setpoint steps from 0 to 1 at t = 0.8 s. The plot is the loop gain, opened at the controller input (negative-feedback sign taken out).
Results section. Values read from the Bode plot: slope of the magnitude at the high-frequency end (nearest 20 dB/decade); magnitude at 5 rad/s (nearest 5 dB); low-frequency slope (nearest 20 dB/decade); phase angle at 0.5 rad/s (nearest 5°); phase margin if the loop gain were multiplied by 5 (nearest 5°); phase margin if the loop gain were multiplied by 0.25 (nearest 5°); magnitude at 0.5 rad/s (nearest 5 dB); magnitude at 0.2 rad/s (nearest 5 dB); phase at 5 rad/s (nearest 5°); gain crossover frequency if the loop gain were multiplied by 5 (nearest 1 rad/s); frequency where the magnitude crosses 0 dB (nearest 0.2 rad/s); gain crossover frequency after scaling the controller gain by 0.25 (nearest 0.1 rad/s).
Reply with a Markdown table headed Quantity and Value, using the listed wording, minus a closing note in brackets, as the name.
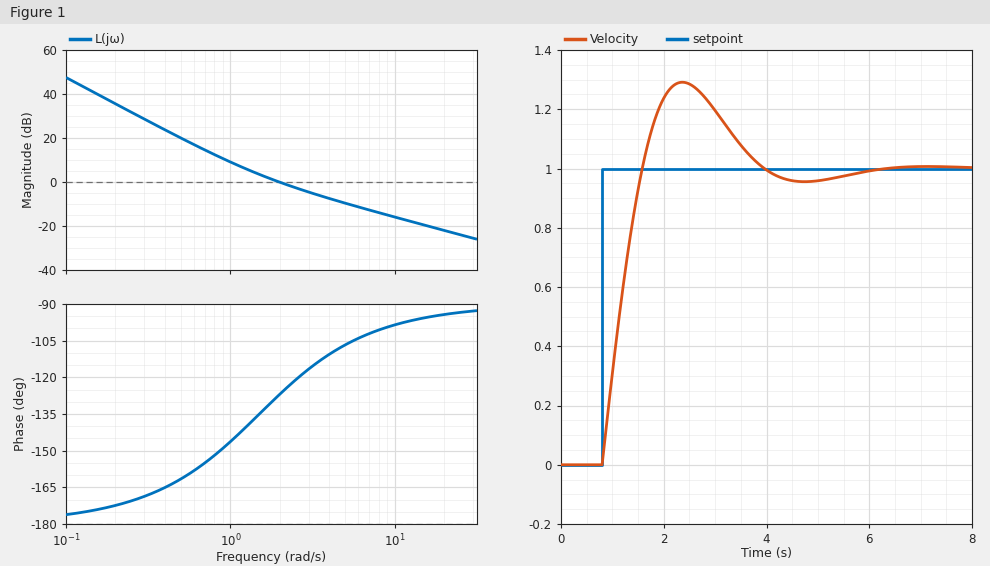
| Quantity | Value |
|---|---|
| slope of the magnitude at the high-frequency end | -20 dB/decade |
| magnitude at 5 rad/s | -10 dB |
| low-frequency slope | -40 dB/decade |
| phase angle at 0.5 rad/s | -160° |
| phase margin if the loop gain were multiplied by 5 | 80° |
| phase margin if the loop gain were multiplied by 0.25 | 30° |
| magnitude at 0.5 rad/s | 20 dB |
| magnitude at 0.2 rad/s | 35 dB |
| phase at 5 rad/s | -105° |
| gain crossover frequency if the loop gain were multiplied by 5 | 8 rad/s |
| frequency where the magnitude crosses 0 dB | 2.0 rad/s |
| gain crossover frequency after scaling the controller gain by 0.25 | 0.8 rad/s |
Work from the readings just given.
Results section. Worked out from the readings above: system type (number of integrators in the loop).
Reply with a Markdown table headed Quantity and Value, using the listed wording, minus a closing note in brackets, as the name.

| Quantity | Value |
|---|---|
| system type | 2 |
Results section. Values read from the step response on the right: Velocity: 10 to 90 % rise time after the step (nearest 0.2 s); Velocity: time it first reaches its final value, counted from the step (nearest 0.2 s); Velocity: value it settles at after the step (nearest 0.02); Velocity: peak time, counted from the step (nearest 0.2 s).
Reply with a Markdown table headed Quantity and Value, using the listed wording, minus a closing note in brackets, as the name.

| Quantity | Value |
|---|---|
| Velocity: 10 to 90 % rise time after the step | 0.6 s |
| Velocity: time it first reaches its final value, counted from the step | 0.8 s |
| Velocity: value it settles at after the step | 1.00 |
| Velocity: peak time, counted from the step | 1.6 s |
